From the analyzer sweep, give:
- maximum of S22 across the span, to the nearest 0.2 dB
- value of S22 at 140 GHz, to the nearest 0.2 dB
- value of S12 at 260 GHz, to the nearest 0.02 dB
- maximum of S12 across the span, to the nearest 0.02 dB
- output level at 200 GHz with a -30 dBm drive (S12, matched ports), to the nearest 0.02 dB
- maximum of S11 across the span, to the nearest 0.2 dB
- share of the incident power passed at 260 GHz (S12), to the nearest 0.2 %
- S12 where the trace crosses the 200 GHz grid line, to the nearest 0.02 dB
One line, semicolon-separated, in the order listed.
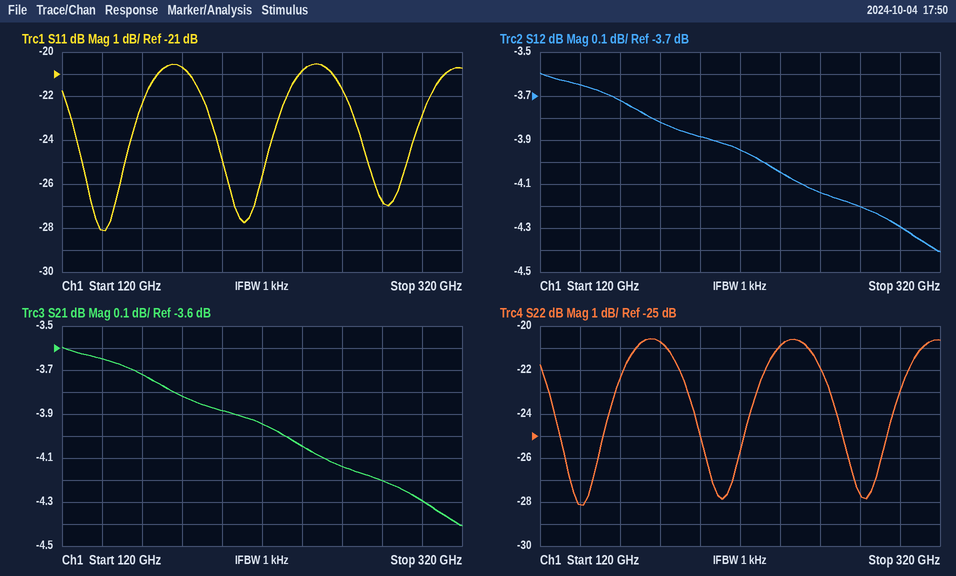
-20.6 dB; -28.2 dB; -4.14 dB; -3.60 dB; -33.88 dBm; -20.6 dB; 38.6 %; -3.88 dB
